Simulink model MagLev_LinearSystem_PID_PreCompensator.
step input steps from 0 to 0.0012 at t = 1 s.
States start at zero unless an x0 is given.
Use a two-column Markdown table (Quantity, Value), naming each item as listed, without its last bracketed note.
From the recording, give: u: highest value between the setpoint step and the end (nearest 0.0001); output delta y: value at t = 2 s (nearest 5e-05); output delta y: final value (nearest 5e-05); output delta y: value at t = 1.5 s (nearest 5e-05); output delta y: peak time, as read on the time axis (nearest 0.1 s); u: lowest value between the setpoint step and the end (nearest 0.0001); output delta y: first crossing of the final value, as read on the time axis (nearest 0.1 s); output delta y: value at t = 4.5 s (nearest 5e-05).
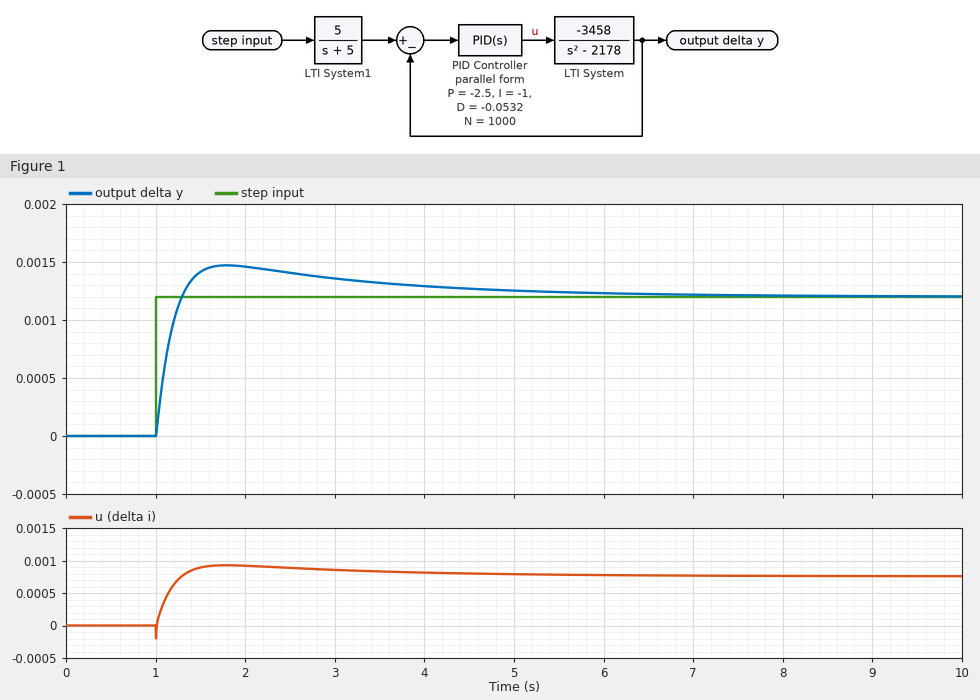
| Quantity | Value |
|---|---|
| u: highest value between the setpoint step and the end | 0.0009 |
| output delta y: value at t = 2 s | 0.00145 |
| output delta y: final value | 0.00120 |
| output delta y: value at t = 1.5 s | 0.00140 |
| output delta y: peak time, as read on the time axis | 1.8 s |
| u: lowest value between the setpoint step and the end | -0.0002 |
| output delta y: first crossing of the final value, as read on the time axis | 1.3 s |
| output delta y: value at t = 4.5 s | 0.00125 |
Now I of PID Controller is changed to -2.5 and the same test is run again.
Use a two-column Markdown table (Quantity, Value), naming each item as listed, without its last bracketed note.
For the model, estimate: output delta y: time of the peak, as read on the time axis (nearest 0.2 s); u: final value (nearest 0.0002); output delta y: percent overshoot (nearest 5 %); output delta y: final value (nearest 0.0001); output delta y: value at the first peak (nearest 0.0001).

| Quantity | Value |
|---|---|
| output delta y: time of the peak, as read on the time axis | 1.6 s |
| u: final value | 0.0008 |
| output delta y: percent overshoot | 15 % |
| output delta y: final value | 0.0012 |
| output delta y: value at the first peak | 0.0014 |
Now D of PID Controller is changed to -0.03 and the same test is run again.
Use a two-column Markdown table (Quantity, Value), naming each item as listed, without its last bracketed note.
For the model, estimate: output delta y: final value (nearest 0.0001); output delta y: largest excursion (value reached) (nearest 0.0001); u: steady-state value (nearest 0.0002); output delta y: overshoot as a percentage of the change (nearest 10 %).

| Quantity | Value |
|---|---|
| output delta y: final value | 0.0012 |
| output delta y: largest excursion (value reached) | 0.0015 |
| u: steady-state value | 0.0008 |
| output delta y: overshoot as a percentage of the change | 20 % |
